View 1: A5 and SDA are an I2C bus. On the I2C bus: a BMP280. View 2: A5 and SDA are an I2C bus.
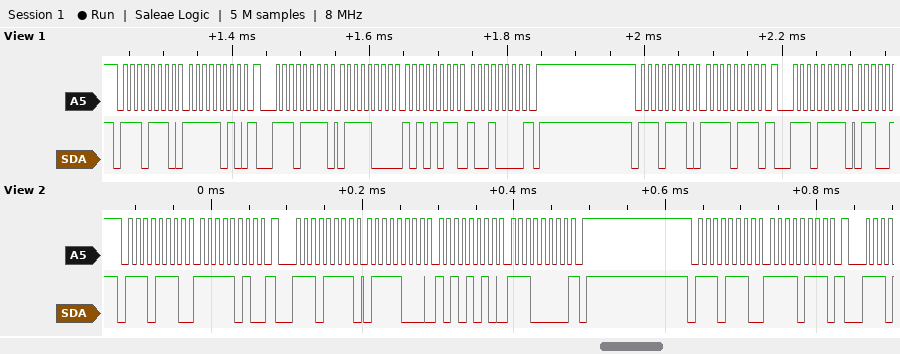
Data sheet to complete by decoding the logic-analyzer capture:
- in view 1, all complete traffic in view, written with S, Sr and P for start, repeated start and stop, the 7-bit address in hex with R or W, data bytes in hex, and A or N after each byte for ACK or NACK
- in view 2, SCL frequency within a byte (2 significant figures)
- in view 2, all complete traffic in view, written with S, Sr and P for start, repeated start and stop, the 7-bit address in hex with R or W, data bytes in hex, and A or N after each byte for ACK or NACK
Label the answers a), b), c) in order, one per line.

a) S 77W A FA A Sr 77R A 78 A AB A 90 N P S 77W A F7 A Sr 77R A
b) 100 kHz
c) S 77W A FA A Sr 77R A 78 A AA A E0 N P S 77W A F7 A
